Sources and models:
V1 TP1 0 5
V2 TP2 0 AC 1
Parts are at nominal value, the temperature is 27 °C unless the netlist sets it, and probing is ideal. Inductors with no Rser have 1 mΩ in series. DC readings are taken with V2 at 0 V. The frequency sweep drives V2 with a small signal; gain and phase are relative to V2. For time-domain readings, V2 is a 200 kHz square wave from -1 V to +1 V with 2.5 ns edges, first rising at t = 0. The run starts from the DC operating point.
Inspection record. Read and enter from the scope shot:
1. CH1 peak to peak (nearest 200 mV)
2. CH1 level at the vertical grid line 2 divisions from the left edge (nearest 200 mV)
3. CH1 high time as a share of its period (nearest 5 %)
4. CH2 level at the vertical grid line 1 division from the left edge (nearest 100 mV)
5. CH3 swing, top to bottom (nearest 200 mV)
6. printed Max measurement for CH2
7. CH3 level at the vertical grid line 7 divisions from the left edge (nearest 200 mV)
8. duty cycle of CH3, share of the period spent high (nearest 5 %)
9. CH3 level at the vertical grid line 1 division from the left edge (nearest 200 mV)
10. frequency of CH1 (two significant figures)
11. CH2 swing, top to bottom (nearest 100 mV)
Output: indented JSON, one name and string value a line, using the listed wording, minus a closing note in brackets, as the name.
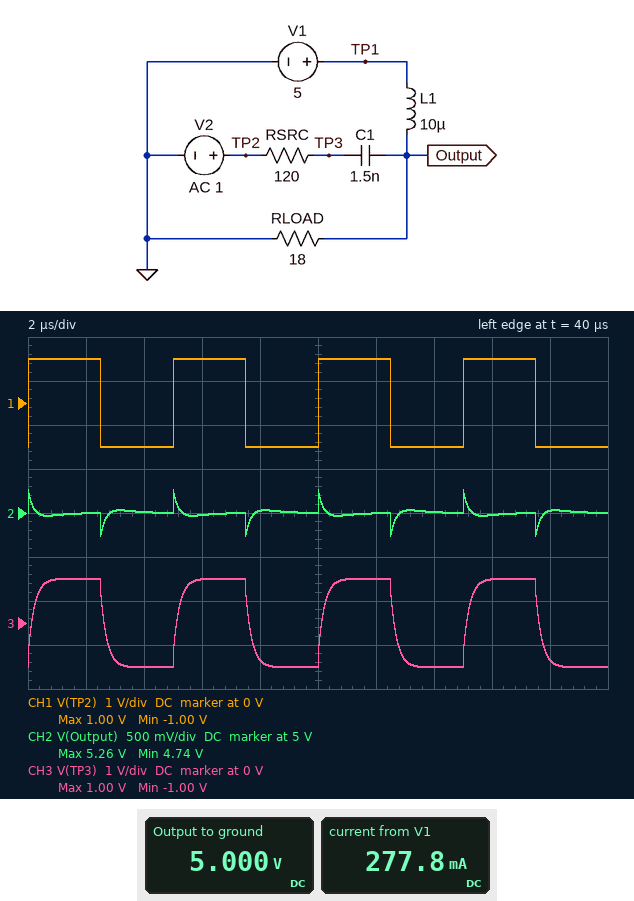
{
  "CH1 peak to peak": "2.0 V",
  "CH1 level at the vertical grid line 2 divisions from the left edge": "-1.0 V",
  "CH1 high time as a share of its period": "50 %",
  "CH2 level at the vertical grid line 1 division from the left edge": "5.0 V",
  "CH3 swing, top to bottom": "2.0 V",
  "printed Max measurement for CH2": "5.26 V",
  "CH3 level at the vertical grid line 7 divisions from the left edge": "-1.0 V",
  "duty cycle of CH3, share of the period spent high": "50 %",
  "CH3 level at the vertical grid line 1 division from the left edge": "1.0 V",
  "frequency of CH1": "200 kHz",
  "CH2 swing, top to bottom": "500 mV"
}
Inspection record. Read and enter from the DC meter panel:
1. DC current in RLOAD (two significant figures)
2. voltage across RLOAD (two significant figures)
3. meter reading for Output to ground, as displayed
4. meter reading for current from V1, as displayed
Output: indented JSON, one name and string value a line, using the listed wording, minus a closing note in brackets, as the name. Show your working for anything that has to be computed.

{
  "DC current in RLOAD": "(5 V) / 18 Ω = 280 mA",
  "voltage across RLOAD": "5 V = 5.0 V",
  "meter reading for Output to ground, as displayed": "5.000 V",
  "meter reading for current from V1, as displayed": "277.8 mA"
}
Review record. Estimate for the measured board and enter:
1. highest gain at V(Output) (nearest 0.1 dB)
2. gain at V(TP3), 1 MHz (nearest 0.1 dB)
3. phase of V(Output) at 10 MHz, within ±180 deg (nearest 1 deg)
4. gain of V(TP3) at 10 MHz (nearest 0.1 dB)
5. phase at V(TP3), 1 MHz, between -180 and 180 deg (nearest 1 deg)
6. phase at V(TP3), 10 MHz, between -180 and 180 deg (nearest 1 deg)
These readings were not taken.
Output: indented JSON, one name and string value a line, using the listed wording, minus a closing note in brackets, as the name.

{
  "highest gain at V(Output)": "-17.7 dB",
  "gain at V(TP3), 1 MHz": "-4.4 dB",
  "phase of V(Output) at 10 MHz, within ±180 deg": "6 deg",
  "gain of V(TP3) at 10 MHz": "-16.5 dB",
  "phase at V(TP3), 1 MHz, between -180 and 180 deg": "-44 deg",
  "phase at V(TP3), 10 MHz, between -180 and 180 deg": "-25 deg"
}
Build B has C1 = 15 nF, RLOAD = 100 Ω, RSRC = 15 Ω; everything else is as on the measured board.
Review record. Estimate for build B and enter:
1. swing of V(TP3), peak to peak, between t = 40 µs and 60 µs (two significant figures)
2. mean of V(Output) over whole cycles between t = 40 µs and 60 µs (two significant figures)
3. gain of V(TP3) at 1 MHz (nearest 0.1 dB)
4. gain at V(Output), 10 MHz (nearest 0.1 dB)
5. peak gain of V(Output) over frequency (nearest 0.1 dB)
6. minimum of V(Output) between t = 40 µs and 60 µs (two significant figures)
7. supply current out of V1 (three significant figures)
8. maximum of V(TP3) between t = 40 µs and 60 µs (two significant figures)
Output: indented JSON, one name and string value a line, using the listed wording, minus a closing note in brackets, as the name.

{
  "swing of V(TP3), peak to peak, between t = 40 µs and 60 µs": "2.3 V",
  "mean of V(Output) over whole cycles between t = 40 µs and 60 µs": "5.0 V",
  "gain of V(TP3) at 1 MHz": "-1.9 dB",
  "gain at V(Output), 10 MHz": "-1.2 dB",
  "peak gain of V(Output) over frequency": "1.6 dB",
  "minimum of V(Output) between t = 40 µs and 60 µs": "3.4 V",
  "supply current out of V1": "50.0 mA",
  "maximum of V(TP3) between t = 40 µs and 60 µs": "1.2 V"
}
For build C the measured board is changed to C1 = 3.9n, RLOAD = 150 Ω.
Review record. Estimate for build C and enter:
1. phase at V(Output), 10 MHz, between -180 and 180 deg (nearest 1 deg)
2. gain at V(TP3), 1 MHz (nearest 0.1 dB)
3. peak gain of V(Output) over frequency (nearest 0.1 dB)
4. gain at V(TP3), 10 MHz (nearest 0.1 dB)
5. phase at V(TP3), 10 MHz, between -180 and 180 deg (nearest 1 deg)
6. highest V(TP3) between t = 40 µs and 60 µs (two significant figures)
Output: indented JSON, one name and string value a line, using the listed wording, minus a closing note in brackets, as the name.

{
  "phase at V(Output), 10 MHz, between -180 and 180 deg": "7 deg",
  "gain at V(TP3), 1 MHz": "-14.9 dB",
  "peak gain of V(Output) over frequency": "-5.1 dB",
  "gain at V(TP3), 10 MHz": "-5.2 dB",
  "phase at V(TP3), 10 MHz, between -180 and 180 deg": "5 deg",
  "highest V(TP3) between t = 40 µs and 60 µs": "1.0 V"
}
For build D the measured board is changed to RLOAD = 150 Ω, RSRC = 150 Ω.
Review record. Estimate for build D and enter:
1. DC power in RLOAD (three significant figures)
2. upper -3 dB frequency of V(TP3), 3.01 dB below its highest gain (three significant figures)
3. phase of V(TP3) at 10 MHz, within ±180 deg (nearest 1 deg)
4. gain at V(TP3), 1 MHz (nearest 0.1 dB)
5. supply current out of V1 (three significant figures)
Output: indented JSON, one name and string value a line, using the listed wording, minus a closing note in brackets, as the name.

{
  "DC power in RLOAD": "167 mW",
  "upper -3 dB frequency of V(TP3), 3.01 dB below its highest gain": "557 kHz",
  "phase of V(TP3) at 10 MHz, within ±180 deg": "5 deg",
  "gain at V(TP3), 1 MHz": "-10.0 dB",
  "supply current out of V1": "33.3 mA"
}
